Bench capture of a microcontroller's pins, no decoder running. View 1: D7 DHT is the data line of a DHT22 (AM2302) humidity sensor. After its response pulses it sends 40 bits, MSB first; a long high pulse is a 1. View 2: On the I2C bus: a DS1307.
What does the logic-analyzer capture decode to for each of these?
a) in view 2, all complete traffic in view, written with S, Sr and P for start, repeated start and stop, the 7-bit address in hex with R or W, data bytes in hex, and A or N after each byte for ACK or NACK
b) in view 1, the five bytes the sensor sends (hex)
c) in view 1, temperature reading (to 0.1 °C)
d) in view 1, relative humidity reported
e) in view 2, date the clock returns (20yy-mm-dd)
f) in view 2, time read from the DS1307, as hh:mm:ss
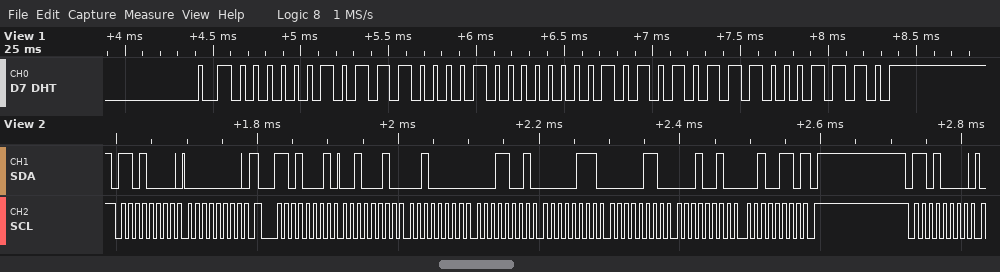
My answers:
S 68W A 00 A Sr 68R A 22 A 20 A 19 A 07 A 06 A 12 A 26 N P S 68W A
02 E1 00 AB 8E
17.1 °C
73.7 %
2026-12-06
19:20:22
